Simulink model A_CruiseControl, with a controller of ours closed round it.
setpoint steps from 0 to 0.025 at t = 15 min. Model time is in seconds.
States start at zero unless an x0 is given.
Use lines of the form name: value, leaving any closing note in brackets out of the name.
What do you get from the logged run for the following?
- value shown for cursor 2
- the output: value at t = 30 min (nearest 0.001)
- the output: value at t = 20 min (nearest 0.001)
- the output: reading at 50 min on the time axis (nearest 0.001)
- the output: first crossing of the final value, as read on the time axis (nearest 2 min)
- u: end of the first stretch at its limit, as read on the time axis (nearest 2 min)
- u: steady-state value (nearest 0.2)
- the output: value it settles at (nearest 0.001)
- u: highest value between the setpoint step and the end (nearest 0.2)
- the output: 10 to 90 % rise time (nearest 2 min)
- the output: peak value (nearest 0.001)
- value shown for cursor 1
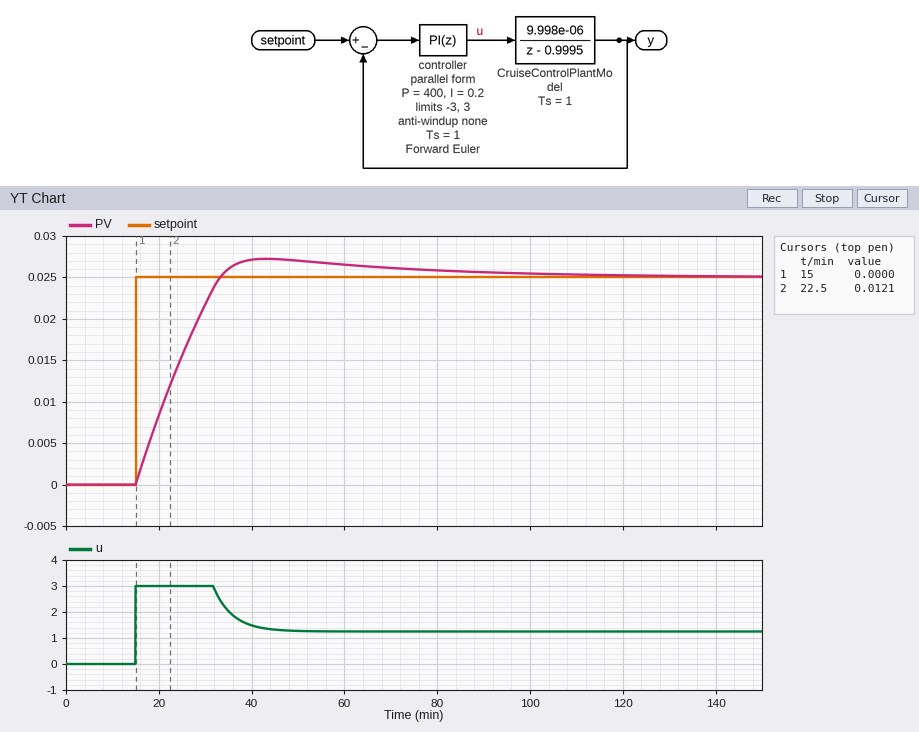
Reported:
value shown for cursor 2: 0.0121
the output: value at t = 30 min: 0.022
the output: value at t = 20 min: 0.008
the output: reading at 50 min on the time axis: 0.027
the output: first crossing of the final value, as read on the time axis: 34 min
u: end of the first stretch at its limit, as read on the time axis: 32 min
u: steady-state value: 1.2
the output: value it settles at: 0.025
u: highest value between the setpoint step and the end: 3.0
the output: 10 to 90 % rise time: 14 min
the output: peak value: 0.027
value shown for cursor 1: 0.0000
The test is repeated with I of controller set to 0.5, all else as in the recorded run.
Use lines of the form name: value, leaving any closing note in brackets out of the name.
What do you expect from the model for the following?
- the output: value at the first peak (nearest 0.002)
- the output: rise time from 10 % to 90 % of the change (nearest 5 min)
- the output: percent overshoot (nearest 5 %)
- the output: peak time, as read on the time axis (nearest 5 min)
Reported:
the output: value at the first peak: 0.032
the output: rise time from 10 % to 90 % of the change: 15 min
the output: percent overshoot: 30 %
the output: peak time, as read on the time axis: 45 min
